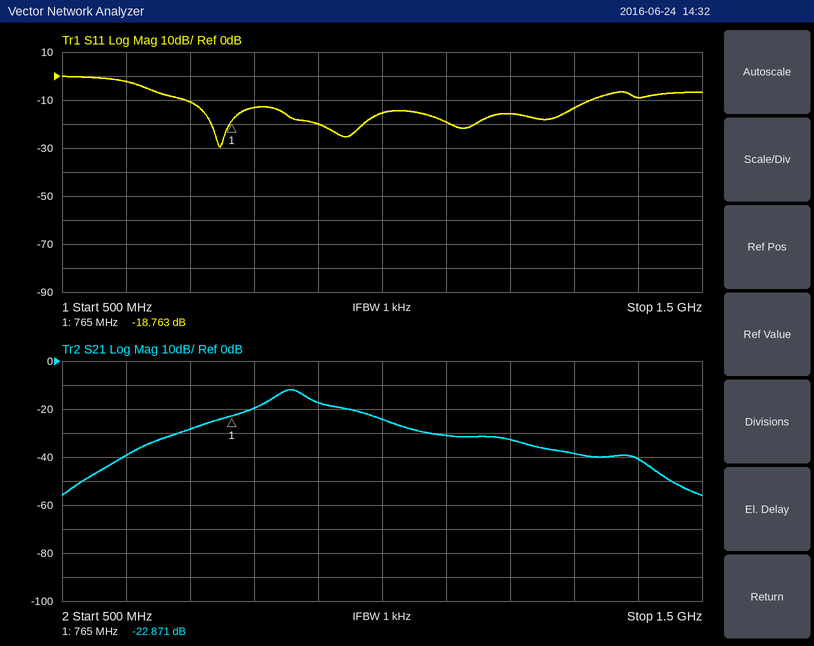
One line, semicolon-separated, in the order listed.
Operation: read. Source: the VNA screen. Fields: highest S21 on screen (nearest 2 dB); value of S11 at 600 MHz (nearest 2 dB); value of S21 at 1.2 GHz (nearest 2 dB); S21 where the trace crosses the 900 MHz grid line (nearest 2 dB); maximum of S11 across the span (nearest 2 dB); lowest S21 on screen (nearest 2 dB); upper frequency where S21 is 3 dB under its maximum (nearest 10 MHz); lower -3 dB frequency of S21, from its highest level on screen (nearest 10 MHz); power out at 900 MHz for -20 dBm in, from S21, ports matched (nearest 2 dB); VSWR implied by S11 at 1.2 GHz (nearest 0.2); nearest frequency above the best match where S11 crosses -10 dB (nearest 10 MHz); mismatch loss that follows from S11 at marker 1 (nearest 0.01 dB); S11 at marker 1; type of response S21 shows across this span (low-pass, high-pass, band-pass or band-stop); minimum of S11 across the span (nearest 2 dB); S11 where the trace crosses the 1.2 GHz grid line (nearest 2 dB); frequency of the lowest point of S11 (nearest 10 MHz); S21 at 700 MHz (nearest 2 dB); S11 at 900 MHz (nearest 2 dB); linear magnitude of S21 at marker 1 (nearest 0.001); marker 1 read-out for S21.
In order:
-12 dB; -2 dB; -32 dB; -18 dB; 0 dB; -56 dB; 880 MHz; 830 MHz; -38 dBm; 1.4; 1.33 GHz; 0.06 dB; -18.763 dB; band-pass; -30 dB; -16 dB; 750 MHz; -28 dB; -20 dB; 0.072; -22.871 dB
